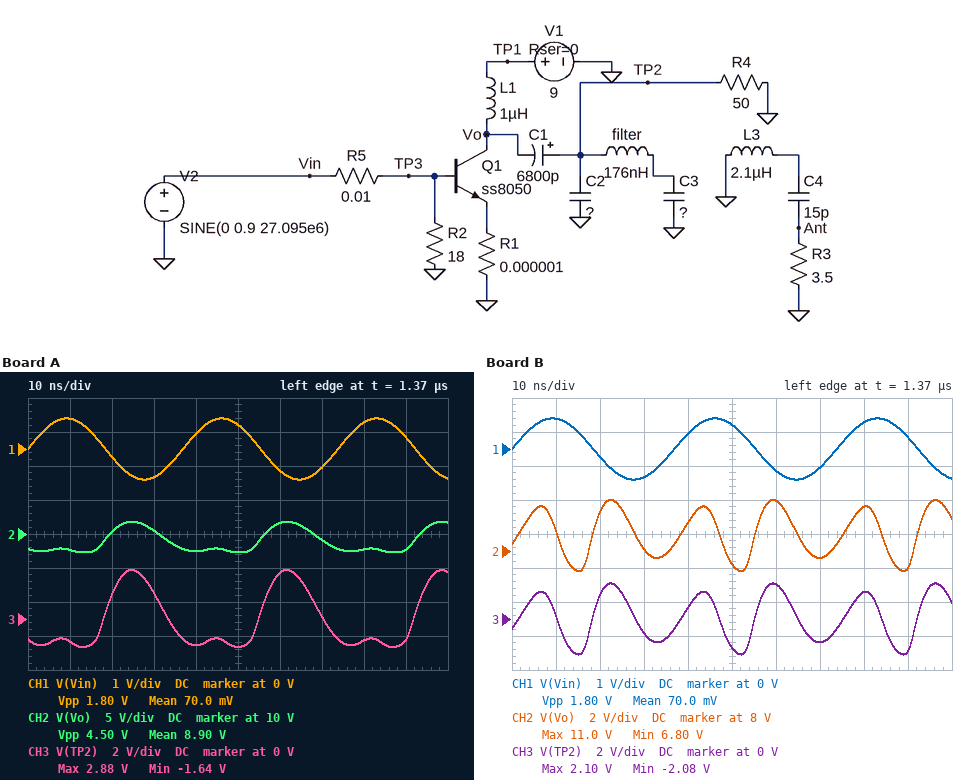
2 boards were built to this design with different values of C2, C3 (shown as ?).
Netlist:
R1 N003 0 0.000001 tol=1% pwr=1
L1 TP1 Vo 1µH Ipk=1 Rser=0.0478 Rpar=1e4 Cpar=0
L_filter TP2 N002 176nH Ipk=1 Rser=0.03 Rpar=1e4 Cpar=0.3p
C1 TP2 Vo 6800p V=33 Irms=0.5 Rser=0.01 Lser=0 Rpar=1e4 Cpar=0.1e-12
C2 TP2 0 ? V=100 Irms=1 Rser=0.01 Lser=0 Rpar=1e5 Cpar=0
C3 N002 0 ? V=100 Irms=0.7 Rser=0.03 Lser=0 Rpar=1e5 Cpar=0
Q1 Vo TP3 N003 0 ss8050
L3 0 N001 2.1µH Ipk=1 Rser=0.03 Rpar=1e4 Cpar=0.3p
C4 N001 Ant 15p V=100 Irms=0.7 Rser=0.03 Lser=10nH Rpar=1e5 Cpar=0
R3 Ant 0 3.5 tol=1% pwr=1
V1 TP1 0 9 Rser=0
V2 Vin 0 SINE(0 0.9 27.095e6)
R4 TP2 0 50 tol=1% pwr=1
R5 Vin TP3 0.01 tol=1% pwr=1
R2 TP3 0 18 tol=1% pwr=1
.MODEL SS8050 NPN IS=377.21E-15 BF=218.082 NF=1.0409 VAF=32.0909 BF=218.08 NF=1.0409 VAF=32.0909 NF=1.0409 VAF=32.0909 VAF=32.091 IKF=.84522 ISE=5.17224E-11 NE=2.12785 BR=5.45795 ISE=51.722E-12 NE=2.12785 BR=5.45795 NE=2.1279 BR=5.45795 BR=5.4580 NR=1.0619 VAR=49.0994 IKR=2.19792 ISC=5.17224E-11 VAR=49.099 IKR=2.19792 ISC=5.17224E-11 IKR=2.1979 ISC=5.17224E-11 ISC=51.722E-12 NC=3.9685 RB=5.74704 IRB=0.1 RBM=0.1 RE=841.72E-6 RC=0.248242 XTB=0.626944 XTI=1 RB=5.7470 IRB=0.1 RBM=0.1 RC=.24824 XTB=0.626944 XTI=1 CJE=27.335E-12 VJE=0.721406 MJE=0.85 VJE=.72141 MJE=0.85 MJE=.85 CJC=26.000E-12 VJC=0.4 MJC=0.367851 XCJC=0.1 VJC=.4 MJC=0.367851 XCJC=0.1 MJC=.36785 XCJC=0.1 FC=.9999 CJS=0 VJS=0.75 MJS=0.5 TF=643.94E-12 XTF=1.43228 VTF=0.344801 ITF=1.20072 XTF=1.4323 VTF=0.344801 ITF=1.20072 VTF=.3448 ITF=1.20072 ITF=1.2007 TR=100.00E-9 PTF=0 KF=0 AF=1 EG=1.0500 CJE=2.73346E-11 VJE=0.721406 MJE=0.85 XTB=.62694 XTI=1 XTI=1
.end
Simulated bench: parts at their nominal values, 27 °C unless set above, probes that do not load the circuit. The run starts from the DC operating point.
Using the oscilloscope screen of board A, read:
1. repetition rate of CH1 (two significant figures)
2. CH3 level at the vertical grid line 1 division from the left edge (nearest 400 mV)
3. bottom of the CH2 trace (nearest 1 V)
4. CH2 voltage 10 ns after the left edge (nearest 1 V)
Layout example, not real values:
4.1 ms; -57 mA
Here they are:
27 MHz; -1.2 V; 7 V; 8 V
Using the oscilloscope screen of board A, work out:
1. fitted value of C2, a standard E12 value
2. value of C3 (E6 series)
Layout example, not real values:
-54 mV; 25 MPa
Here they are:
220 pF; 470 pF
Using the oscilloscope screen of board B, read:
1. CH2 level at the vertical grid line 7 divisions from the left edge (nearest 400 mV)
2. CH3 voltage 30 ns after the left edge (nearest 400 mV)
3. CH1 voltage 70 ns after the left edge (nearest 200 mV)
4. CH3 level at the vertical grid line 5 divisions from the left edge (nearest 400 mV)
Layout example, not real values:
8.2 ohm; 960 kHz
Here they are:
7.6 V; -800 mV; -600 mV; -1.6 V
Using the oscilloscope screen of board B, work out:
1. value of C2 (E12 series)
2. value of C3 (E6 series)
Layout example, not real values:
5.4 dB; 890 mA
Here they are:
120 pF; 220 pF
